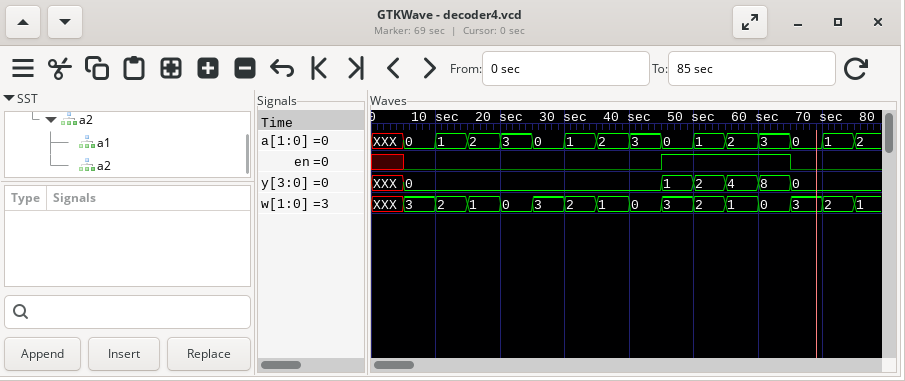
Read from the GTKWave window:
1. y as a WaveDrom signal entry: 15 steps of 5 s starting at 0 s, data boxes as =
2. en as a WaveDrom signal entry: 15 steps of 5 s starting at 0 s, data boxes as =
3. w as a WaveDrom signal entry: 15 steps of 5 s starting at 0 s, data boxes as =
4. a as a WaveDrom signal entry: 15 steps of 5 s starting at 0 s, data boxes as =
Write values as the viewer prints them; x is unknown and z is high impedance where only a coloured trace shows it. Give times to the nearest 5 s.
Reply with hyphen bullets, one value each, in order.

- {name: 'y', wave: 'x=.......=====.', data: '0 1 2 4 8 0'}
- {name: 'en', wave: 'x0.......1...0.'}
- {name: 'w', wave: 'x==============', data: '3 2 1 0 3 2 1 0 3 2 1 0 3 2'}
- {name: 'a', wave: 'x==============', data: '0 1 2 3 0 1 2 3 0 1 2 3 0 1'}
